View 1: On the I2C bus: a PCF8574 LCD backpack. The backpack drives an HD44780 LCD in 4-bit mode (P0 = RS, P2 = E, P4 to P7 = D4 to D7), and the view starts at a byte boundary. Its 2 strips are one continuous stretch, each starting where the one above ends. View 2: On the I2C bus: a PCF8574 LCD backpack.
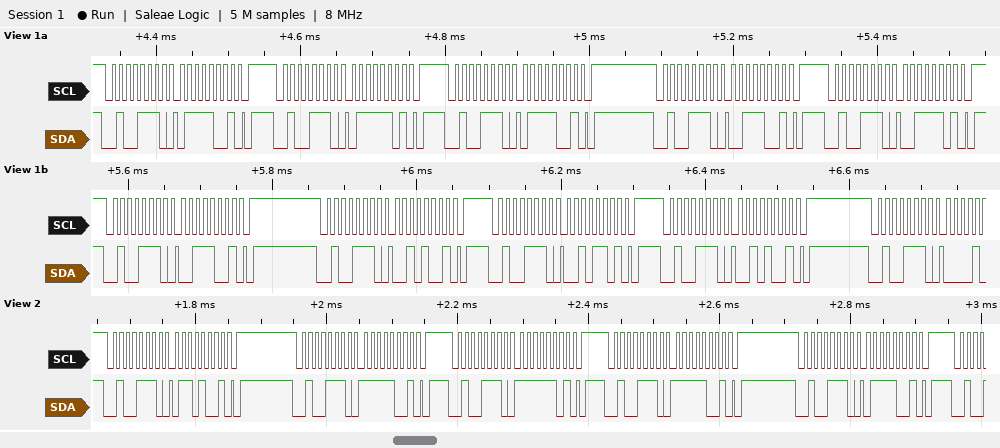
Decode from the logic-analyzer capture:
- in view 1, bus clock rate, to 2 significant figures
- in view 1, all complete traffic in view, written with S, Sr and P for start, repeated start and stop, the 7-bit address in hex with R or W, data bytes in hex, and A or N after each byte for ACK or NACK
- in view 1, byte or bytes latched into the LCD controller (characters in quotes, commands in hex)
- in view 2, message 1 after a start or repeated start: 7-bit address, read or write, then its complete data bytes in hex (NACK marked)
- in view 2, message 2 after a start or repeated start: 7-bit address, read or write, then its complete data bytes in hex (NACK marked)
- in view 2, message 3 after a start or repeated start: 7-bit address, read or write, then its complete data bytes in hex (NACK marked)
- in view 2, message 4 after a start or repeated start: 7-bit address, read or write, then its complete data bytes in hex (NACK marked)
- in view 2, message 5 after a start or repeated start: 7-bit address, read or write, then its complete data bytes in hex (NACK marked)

100 kHz
S 27W A 79 A P S 27W A 7D A P S 27W A 79 A P S 27W A 39 A P S 27W A 3D A P S 27W A 39 A P S 27W A 29 A P S 27W A 2D A P S 27W A 29 A P S 27W A
's'
0x27 write: 69
0x27 write: F9
0x27 write: FD
0x27 write: F9
0x27 write: 79
